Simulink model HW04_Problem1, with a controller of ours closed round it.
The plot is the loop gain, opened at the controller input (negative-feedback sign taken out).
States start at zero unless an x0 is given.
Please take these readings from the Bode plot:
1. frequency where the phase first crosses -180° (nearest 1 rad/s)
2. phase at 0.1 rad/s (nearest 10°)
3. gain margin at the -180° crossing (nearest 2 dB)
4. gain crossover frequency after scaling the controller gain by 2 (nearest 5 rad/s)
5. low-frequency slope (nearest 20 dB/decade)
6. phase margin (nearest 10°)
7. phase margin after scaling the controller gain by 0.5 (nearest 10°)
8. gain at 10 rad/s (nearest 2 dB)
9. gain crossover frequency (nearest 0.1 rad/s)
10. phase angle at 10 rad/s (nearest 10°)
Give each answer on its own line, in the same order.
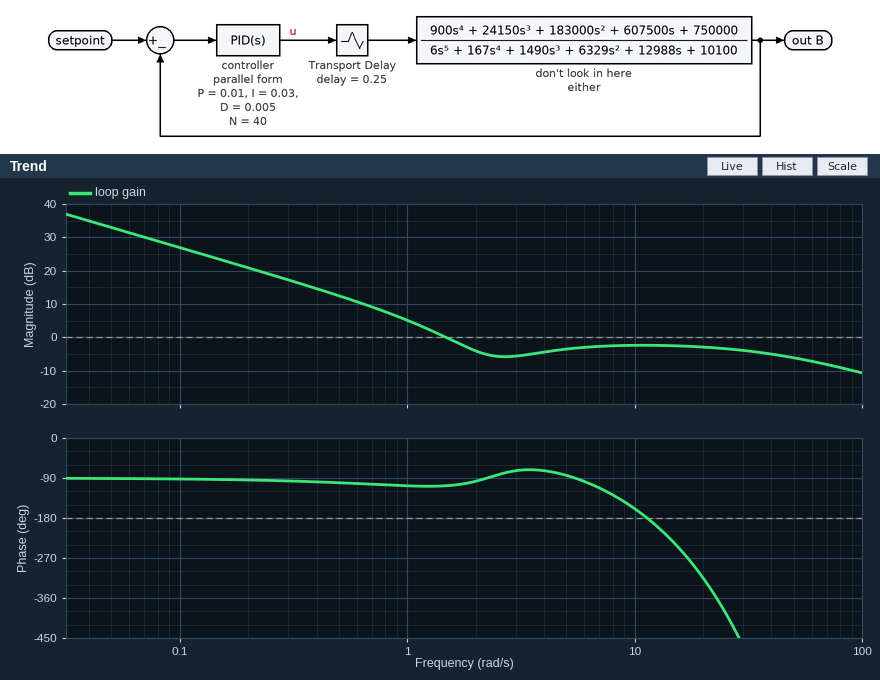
11 rad/s
-90°
2 dB
50 rad/s
-20 dB/decade
70°
70°
-2 dB
1.5 rad/s
-160°
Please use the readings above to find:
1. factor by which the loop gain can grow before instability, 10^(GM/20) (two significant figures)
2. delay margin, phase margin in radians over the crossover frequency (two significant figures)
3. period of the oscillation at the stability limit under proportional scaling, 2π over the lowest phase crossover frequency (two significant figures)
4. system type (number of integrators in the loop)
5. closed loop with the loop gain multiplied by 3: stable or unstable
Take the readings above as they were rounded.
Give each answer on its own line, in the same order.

1.3
0.81 s
0.57 s
1
unstable
